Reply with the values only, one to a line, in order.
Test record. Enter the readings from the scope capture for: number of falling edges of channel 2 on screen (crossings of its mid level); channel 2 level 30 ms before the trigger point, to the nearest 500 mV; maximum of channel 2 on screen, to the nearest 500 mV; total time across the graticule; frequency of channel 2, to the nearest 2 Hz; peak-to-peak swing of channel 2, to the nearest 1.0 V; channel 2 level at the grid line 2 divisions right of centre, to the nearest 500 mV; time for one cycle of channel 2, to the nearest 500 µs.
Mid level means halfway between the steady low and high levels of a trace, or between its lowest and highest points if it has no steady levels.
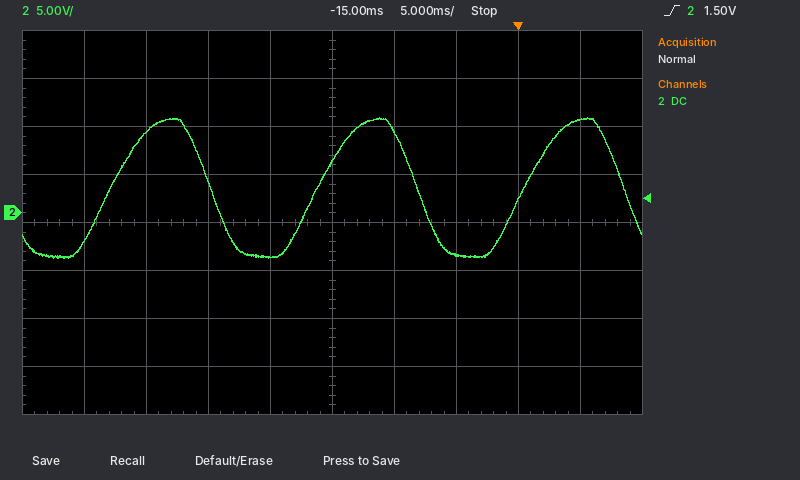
3
8.5 V
10.0 V
50 ms
60 Hz
15.0 V
-4.5 V
16.5 ms
